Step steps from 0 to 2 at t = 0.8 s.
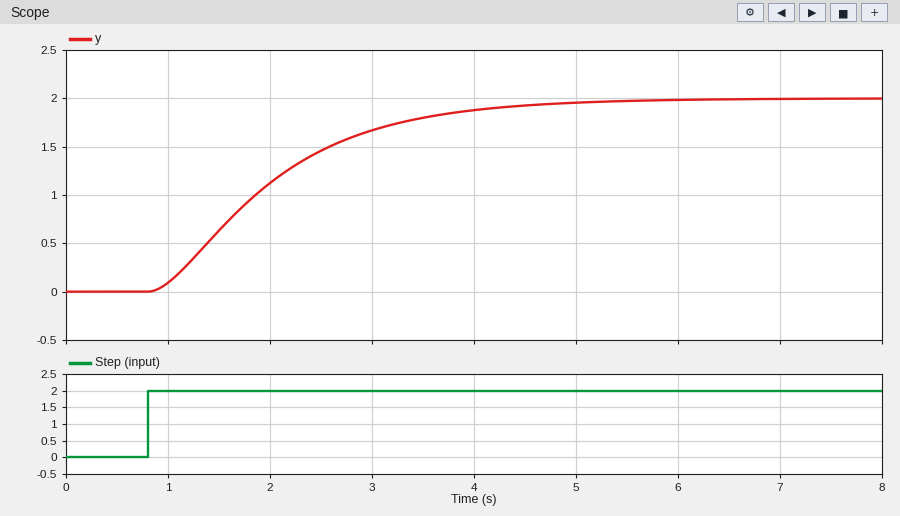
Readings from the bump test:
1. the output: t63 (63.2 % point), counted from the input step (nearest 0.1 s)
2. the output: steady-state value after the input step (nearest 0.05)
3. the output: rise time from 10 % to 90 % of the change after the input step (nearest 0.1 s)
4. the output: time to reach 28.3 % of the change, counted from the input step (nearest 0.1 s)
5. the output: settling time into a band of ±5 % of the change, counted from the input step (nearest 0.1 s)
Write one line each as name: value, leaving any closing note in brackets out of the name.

the output: t63 (63.2 % point), counted from the input step: 1.4 s
the output: steady-state value after the input step: 2.00
the output: rise time from 10 % to 90 % of the change after the input step: 2.4 s
the output: time to reach 28.3 % of the change, counted from the input step: 0.6 s
the output: settling time into a band of ±5 % of the change, counted from the input step: 3.4 s
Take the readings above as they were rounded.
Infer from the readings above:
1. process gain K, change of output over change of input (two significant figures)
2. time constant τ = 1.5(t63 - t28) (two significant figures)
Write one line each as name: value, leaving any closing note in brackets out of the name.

process gain K, change of output over change of input: 1.0
time constant τ = 1.5(t63 - t28): 1.2 s
